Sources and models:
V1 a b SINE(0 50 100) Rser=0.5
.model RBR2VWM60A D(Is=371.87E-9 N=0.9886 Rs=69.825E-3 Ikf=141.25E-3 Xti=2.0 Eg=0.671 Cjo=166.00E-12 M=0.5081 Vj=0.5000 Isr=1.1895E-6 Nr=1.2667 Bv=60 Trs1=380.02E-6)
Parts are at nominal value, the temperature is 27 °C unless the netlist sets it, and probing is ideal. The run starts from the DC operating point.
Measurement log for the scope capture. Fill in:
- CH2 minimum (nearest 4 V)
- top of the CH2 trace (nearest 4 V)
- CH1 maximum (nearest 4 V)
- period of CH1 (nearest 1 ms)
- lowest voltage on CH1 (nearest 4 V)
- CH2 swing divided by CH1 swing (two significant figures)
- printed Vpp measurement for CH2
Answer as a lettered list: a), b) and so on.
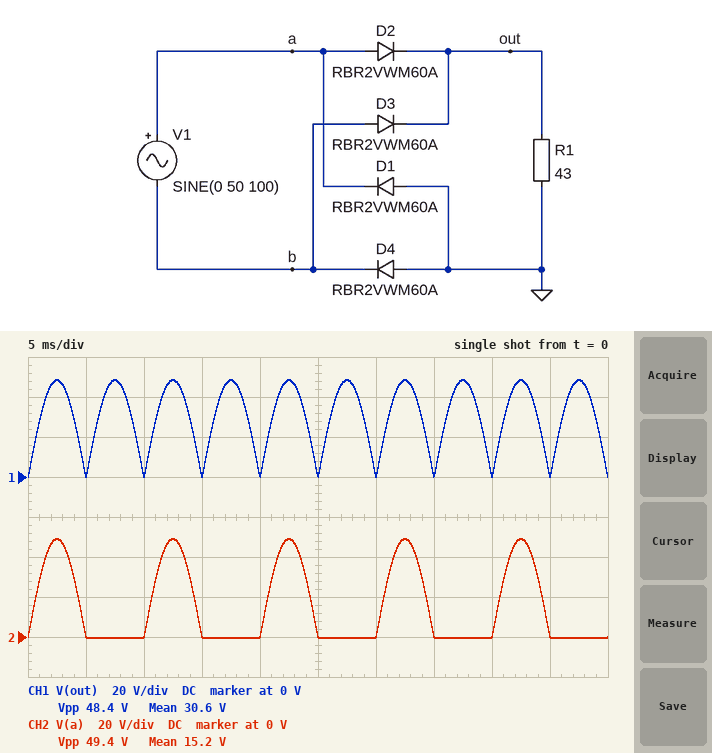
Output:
a) 0 V
b) 48 V
c) 48 V
d) 5 ms
e) 0 V
f) 1.0
g) 49.4 V
